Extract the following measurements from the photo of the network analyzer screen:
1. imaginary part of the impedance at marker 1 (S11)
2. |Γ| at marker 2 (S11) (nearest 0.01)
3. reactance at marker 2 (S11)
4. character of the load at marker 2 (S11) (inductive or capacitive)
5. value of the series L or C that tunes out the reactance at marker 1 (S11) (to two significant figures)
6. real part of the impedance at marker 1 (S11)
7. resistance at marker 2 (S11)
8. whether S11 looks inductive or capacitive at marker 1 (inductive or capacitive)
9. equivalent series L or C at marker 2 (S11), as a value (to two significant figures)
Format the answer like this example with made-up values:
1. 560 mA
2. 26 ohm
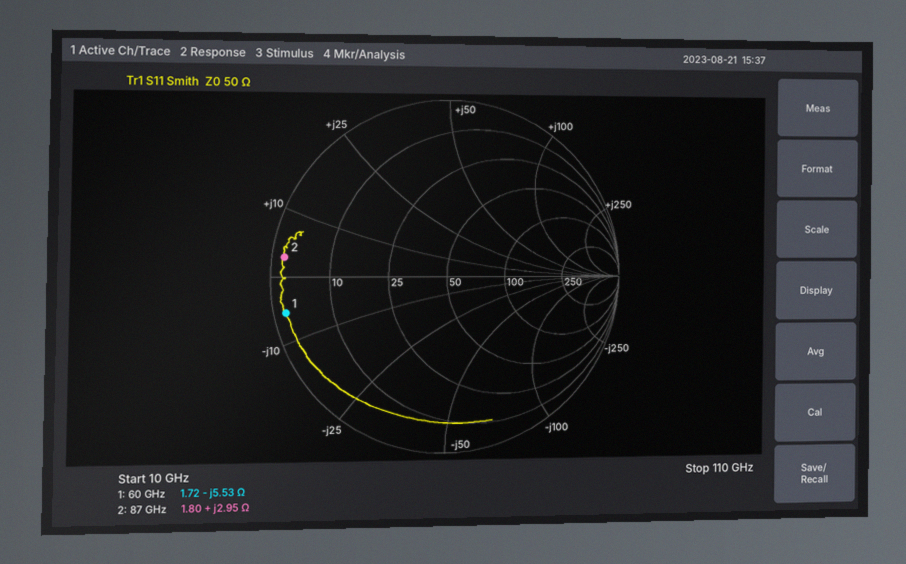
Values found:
1. -5.53 Ω
2. 0.93
3. +2.95 Ω
4. inductive
5. 15 pH
6. 1.72 Ω
7. 1.80 Ω
8. capacitive
9. 5.4 pH
